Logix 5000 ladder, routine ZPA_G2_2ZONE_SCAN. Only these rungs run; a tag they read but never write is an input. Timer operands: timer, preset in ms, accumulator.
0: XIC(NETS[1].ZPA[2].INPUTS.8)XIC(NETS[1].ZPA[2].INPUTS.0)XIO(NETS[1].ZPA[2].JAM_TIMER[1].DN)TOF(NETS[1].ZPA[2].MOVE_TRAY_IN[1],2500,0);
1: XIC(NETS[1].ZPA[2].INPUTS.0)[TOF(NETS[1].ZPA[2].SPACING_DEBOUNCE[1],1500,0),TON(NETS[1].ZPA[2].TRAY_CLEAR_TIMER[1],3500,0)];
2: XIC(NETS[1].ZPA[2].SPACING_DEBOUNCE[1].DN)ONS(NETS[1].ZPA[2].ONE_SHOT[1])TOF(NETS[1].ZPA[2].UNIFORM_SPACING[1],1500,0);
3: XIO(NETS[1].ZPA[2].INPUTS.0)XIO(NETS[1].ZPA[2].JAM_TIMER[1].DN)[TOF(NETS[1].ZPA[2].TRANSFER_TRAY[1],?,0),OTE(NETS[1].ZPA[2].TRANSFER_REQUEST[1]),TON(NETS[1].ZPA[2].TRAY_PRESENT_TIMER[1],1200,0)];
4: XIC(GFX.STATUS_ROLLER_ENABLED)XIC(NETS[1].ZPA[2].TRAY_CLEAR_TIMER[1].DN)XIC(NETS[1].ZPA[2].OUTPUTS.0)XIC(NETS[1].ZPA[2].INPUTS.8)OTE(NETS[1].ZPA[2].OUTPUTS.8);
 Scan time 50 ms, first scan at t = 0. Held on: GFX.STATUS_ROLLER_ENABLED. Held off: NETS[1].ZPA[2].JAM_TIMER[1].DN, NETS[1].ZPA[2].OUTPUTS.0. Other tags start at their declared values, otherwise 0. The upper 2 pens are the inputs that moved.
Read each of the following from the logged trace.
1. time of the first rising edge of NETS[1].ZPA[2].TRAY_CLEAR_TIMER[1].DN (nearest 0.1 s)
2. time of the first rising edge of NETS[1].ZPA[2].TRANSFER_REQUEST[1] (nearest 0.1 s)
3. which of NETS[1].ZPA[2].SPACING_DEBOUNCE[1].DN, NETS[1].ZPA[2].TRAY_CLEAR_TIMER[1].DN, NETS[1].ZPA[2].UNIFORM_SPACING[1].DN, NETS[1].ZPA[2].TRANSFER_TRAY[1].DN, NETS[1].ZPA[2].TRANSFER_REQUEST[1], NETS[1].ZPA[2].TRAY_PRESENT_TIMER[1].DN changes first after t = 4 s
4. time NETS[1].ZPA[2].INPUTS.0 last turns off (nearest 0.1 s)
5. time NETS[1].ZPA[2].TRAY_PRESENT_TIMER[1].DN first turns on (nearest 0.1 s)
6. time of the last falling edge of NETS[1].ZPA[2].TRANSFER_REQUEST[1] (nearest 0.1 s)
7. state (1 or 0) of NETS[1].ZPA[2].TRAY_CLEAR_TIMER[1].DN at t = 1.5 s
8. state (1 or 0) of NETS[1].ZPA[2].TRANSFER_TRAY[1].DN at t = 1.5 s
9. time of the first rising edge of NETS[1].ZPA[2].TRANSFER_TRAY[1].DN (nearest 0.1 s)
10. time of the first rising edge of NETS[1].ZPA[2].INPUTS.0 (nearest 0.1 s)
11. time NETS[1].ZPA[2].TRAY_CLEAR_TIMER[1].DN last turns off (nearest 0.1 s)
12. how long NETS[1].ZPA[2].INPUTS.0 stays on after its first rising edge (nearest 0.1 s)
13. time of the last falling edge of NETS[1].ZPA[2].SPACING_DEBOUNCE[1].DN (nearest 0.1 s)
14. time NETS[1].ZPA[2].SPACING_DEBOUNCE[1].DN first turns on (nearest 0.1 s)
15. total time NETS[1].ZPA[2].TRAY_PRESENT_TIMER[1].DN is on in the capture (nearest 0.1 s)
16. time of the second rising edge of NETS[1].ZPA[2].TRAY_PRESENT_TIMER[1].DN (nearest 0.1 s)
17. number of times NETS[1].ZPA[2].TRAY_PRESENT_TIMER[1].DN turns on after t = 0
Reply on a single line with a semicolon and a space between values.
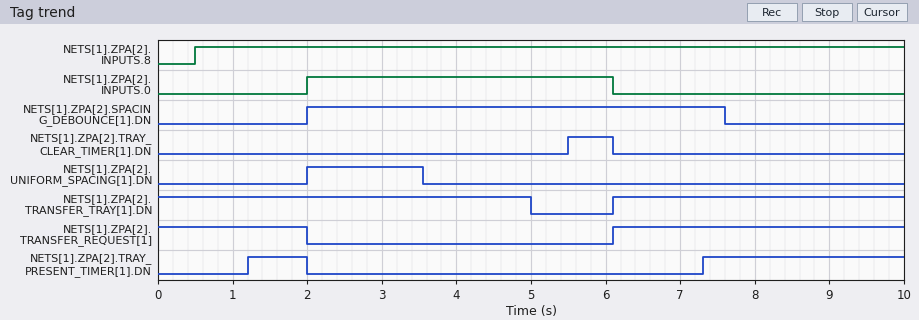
5.5 s; 6.1 s; NETS[1].ZPA[2].TRANSFER_TRAY[1].DN; 6.1 s; 1.2 s; 2.0 s; 0; 1; 6.1 s; 2.0 s; 6.1 s; 4.1 s; 7.6 s; 2.0 s; 3.5 s; 7.3 s; 2
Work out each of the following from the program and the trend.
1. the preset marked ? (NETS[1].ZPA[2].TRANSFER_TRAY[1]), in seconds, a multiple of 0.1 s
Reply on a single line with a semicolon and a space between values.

3.0 s
